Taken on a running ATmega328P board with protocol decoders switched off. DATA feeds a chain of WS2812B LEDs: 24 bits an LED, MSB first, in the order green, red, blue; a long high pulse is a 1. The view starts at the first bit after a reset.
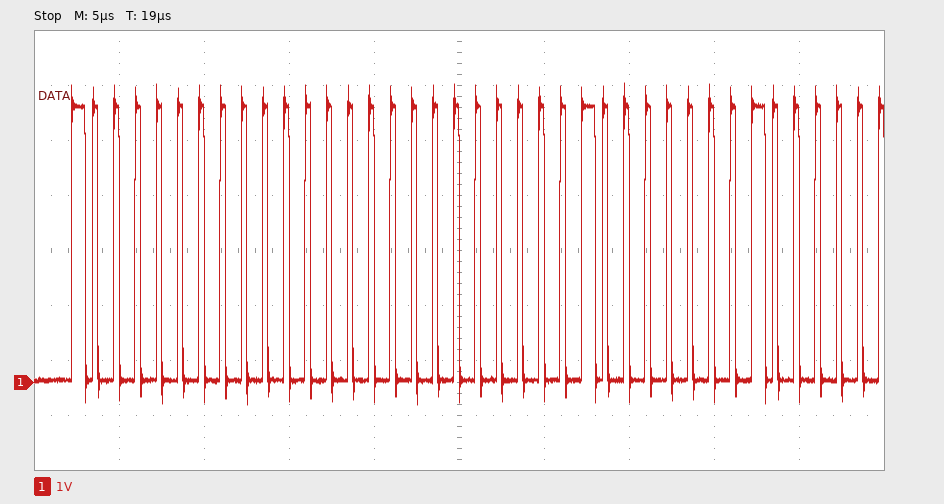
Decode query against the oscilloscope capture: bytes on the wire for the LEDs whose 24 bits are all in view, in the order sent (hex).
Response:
80 00 00
